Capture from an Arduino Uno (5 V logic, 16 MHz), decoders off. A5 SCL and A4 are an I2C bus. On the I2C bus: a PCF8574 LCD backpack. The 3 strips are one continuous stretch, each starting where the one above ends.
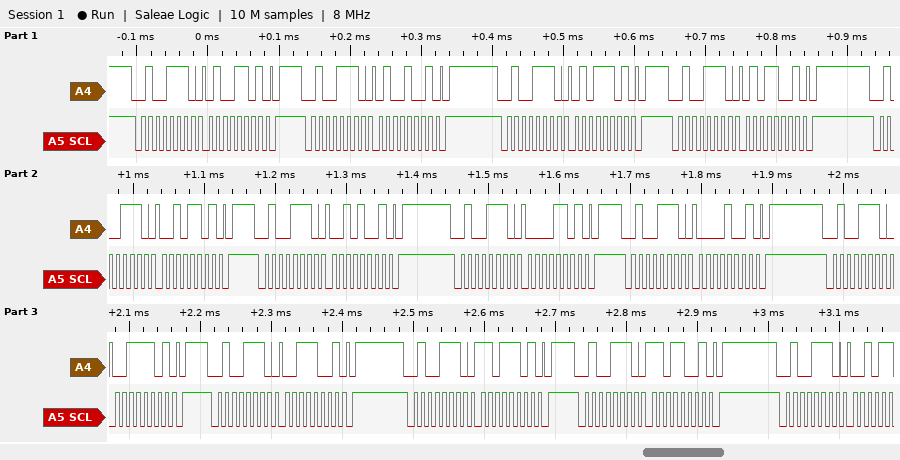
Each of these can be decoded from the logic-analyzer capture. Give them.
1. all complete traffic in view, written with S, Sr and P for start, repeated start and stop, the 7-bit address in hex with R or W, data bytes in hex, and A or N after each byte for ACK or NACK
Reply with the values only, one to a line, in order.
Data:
S 27W A 4D A P S 27W A 49 A P S 27W A 5D A P S 27W A 59 A P S 27W A 2D A P S 27W A 29 A P S 27W A 0D A P S 27W A 09 A P S 27W A 3D A P S 27W A 39 A P S 27W A DD A P S 27W A D9 A P S 27W A
